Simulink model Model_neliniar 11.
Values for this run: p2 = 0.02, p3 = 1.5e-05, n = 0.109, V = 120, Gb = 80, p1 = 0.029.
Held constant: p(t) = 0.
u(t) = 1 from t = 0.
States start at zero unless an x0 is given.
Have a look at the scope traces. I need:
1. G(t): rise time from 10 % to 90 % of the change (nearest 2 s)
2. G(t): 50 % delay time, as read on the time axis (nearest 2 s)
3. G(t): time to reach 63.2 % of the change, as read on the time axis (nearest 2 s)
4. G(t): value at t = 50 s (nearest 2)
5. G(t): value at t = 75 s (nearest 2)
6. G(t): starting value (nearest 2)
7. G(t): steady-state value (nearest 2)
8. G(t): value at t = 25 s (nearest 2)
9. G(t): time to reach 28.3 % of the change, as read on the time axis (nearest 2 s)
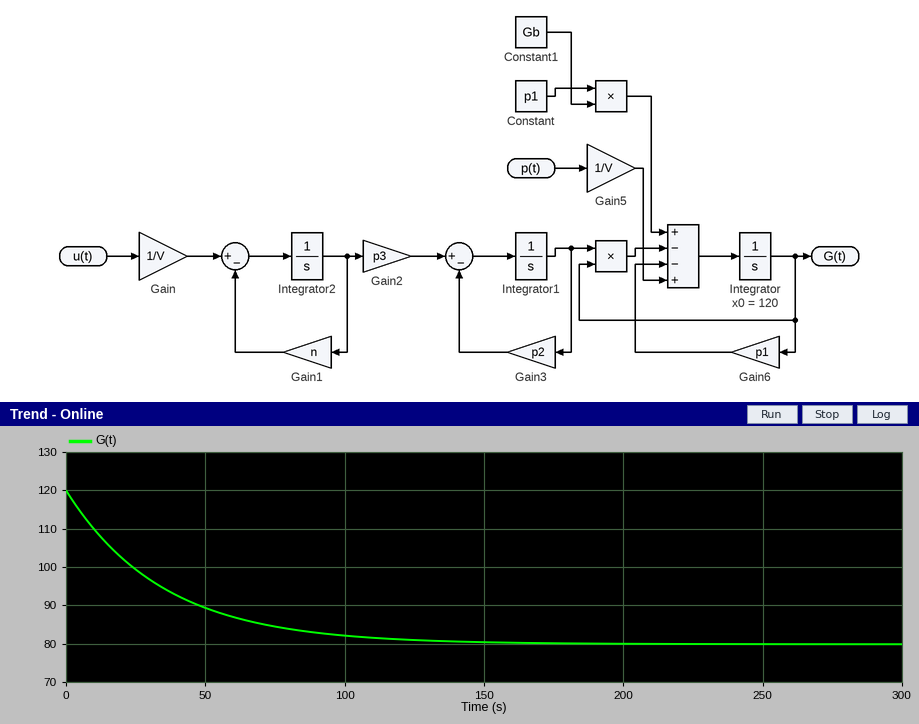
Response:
76 s
24 s
34 s
90
84
120
80
100
12 s
